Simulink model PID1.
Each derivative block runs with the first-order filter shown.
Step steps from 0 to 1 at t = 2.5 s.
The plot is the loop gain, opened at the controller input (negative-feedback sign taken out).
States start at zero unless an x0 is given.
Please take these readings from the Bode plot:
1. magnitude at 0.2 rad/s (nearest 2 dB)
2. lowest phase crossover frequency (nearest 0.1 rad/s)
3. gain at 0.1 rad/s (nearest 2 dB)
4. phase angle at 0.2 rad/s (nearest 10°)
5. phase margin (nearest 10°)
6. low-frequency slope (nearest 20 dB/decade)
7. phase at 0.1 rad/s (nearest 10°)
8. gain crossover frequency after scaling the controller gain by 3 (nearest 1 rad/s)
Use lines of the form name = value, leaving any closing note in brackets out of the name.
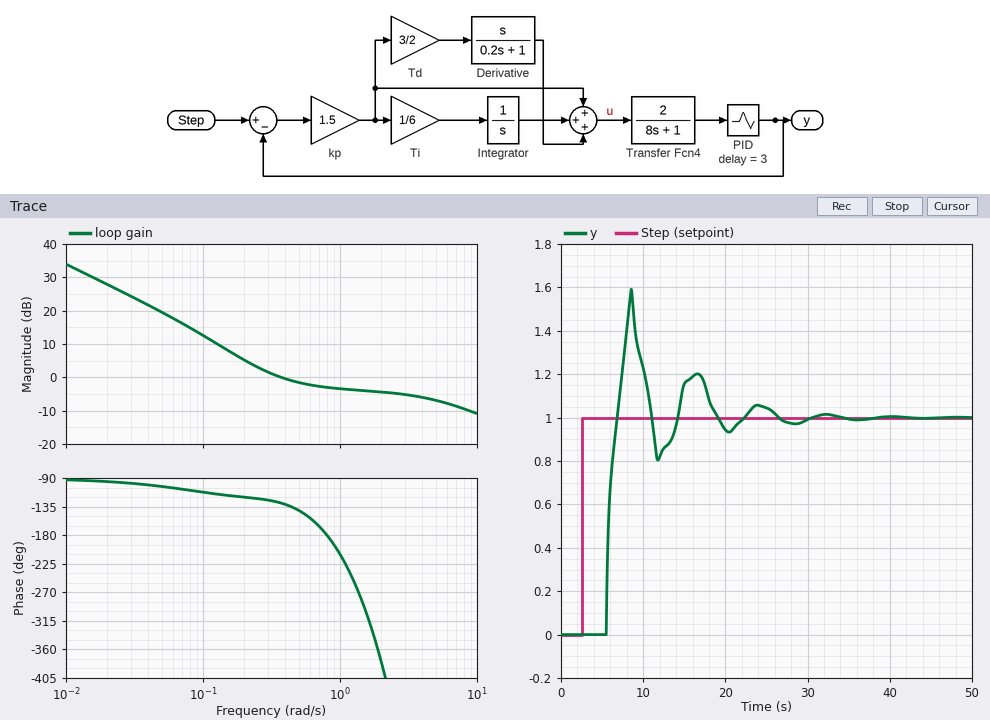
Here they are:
magnitude at 0.2 rad/s = 6 dB
lowest phase crossover frequency = 0.8 rad/s
gain at 0.1 rad/s = 12 dB
phase angle at 0.2 rad/s = -120°
phase margin = 50°
low-frequency slope = -20 dB/decade
phase at 0.1 rad/s = -110°
gain crossover frequency after scaling the controller gain by 3 = 8 rad/s
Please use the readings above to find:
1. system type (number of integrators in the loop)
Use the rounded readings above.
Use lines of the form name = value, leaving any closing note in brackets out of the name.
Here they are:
system type = 1
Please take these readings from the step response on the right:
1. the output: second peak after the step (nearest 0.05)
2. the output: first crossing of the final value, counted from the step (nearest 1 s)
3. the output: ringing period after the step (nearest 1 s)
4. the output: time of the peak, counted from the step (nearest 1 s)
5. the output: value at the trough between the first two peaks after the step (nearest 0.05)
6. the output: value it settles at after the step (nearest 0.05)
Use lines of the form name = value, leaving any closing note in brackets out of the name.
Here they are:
the output: second peak after the step = 1.20
the output: first crossing of the final value, counted from the step = 4 s
the output: ringing period after the step = 8 s
the output: time of the peak, counted from the step = 6 s
the output: value at the trough between the first two peaks after the step = 0.80
the output: value it settles at after the step = 1.00
